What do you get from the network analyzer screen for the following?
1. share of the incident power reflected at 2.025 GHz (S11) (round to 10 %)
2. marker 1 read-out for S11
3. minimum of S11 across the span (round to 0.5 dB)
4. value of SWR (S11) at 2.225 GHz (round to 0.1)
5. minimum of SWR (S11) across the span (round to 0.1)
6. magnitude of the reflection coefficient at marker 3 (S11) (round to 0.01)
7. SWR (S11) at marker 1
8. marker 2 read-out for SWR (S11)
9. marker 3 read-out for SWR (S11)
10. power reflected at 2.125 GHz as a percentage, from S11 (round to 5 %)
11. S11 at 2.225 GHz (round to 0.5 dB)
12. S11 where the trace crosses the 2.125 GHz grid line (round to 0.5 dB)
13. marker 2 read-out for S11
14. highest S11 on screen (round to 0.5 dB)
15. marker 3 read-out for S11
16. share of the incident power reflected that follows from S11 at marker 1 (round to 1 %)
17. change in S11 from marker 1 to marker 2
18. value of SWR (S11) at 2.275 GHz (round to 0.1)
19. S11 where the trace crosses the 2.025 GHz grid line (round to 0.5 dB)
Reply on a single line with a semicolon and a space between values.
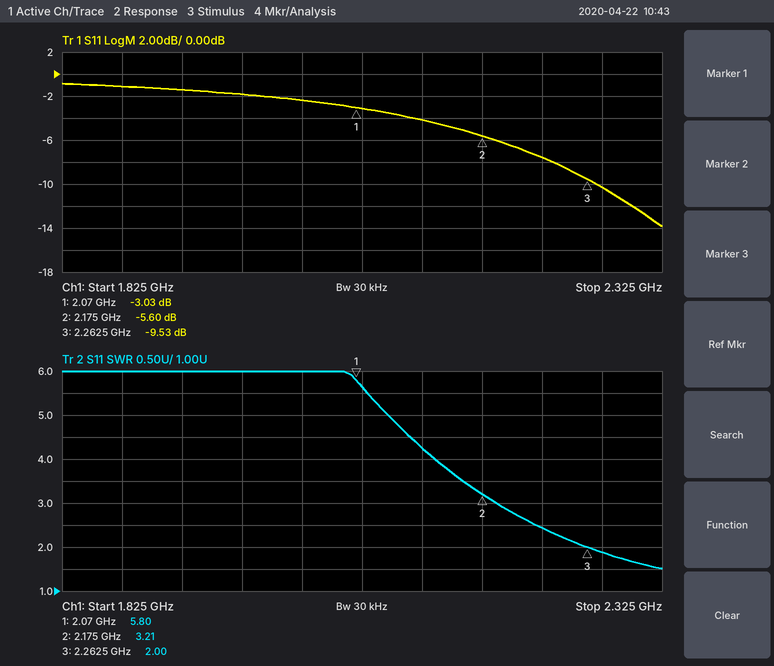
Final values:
60 %; -3.03 dB; -14.0 dB; 2.4; 1.5; 0.33; 5.80; 3.21; 2.00; 40 %; -7.5 dB; -4.0 dB; -5.60 dB; -1.0 dB; -9.53 dB; 50 %; -2.57 dB; 1.9; -2.5 dB
